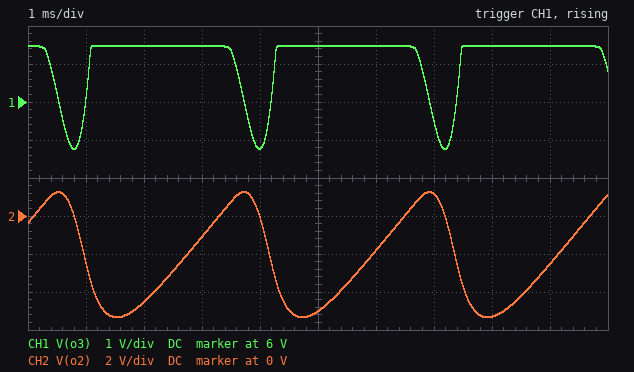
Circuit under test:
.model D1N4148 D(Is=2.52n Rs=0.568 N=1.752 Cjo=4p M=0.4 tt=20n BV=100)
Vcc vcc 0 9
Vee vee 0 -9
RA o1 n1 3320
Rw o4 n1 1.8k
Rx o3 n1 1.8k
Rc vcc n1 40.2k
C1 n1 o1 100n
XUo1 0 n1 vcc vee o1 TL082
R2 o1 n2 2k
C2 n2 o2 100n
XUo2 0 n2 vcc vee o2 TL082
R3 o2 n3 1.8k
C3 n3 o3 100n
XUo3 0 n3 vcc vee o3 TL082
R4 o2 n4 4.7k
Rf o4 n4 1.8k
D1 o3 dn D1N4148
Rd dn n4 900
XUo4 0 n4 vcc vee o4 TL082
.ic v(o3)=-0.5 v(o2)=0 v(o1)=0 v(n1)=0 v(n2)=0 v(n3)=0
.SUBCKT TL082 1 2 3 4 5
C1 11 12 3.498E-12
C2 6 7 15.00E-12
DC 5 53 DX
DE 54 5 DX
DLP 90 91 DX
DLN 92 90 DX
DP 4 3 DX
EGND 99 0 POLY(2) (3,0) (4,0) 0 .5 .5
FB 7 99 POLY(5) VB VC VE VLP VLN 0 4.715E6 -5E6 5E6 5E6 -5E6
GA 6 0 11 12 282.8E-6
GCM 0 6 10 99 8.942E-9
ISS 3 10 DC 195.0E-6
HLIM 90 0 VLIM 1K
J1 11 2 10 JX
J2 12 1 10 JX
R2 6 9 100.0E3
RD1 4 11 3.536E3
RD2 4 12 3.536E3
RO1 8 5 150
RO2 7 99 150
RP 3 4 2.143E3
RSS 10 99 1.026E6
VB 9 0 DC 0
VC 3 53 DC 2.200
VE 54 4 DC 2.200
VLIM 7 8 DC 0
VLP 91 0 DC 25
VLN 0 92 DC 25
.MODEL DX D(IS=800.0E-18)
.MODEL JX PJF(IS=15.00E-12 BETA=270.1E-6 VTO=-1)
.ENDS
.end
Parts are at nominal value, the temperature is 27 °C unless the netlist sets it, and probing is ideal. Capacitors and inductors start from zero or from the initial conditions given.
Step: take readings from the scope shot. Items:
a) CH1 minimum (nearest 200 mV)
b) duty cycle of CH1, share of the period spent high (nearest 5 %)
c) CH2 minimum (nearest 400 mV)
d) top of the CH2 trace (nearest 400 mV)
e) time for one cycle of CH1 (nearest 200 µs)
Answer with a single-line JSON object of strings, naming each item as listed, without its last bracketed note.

{"CH1 minimum": "4.8 V", "duty cycle of CH1, share of the period spent high": "85 %", "CH2 minimum": "-5.2 V", "top of the CH2 trace": "1.2 V", "time for one cycle of CH1": "3.2 ms"}
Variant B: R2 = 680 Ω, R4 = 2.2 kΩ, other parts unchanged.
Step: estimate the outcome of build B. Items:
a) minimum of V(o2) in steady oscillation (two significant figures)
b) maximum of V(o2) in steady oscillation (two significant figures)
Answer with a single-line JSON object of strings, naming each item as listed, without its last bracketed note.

{"minimum of V(o2) in steady oscillation": "-3.2 V", "maximum of V(o2) in steady oscillation": "2.2 V"}
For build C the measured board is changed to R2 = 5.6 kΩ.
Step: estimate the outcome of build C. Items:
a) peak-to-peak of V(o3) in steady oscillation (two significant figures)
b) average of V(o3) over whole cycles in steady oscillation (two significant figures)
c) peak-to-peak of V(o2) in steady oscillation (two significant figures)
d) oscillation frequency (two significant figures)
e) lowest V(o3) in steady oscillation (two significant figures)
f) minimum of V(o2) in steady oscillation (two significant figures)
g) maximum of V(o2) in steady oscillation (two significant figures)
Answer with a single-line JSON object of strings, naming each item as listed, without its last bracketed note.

{"peak-to-peak of V(o3) in steady oscillation": "1.9 V", "average of V(o3) over whole cycles in steady oscillation": "7.1 V", "peak-to-peak of V(o2) in steady oscillation": "2.3 V", "oscillation frequency": "290 Hz", "lowest V(o3) in steady oscillation": "5.6 V", "minimum of V(o2) in steady oscillation": "-1.8 V", "maximum of V(o2) in steady oscillation": "560 mV"}
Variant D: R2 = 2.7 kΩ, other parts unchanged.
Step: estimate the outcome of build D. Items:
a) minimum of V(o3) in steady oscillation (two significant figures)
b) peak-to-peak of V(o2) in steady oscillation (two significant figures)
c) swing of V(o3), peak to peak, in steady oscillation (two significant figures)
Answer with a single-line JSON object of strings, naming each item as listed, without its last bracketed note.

{"minimum of V(o3) in steady oscillation": "5.1 V", "peak-to-peak of V(o2) in steady oscillation": "4.8 V", "swing of V(o3), peak to peak, in steady oscillation": "2.4 V"}
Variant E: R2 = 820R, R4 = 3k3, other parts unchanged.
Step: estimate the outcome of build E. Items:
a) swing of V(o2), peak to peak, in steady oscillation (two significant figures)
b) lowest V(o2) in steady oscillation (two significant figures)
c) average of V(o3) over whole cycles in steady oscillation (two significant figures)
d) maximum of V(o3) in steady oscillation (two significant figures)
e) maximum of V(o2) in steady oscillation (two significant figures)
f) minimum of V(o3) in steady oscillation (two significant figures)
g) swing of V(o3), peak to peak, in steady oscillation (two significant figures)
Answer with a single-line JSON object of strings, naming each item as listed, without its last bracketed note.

{"swing of V(o2), peak to peak, in steady oscillation": "10 V", "lowest V(o2) in steady oscillation": "-7.5 V", "average of V(o3) over whole cycles in steady oscillation": "6.9 V", "maximum of V(o3) in steady oscillation": "7.5 V", "maximum of V(o2) in steady oscillation": "2.5 V", "minimum of V(o3) in steady oscillation": "3.6 V", "swing of V(o3), peak to peak, in steady oscillation": "3.9 V"}
